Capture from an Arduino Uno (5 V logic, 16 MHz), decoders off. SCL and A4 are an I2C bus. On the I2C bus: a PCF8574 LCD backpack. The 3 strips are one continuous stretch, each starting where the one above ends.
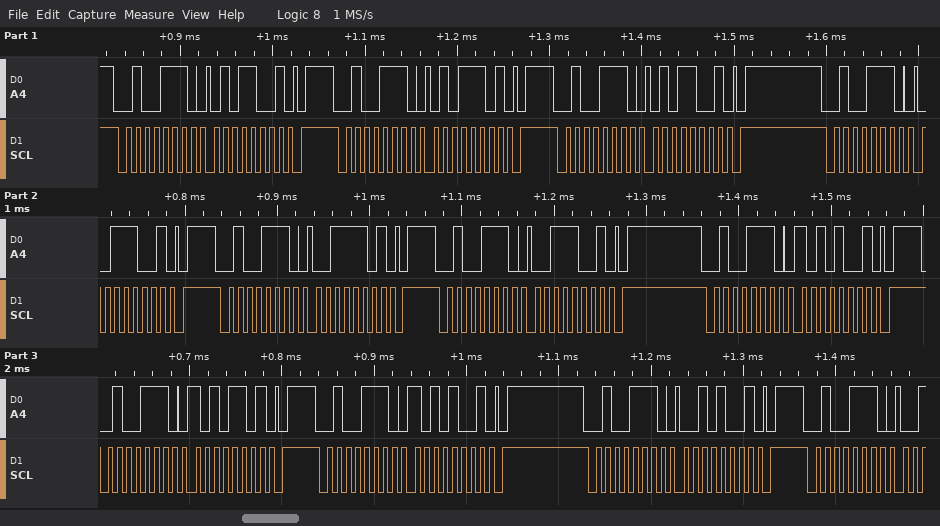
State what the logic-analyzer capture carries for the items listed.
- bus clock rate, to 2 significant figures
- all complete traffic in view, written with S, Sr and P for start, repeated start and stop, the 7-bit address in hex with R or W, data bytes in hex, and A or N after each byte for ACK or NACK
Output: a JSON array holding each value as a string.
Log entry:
["100 kHz", "S 27W A 59 A P S 27W A 5D A P S 27W A 59 A P S 27W A 39 A P S 27W A 3D A P S 27W A 39 A P S 27W A A9 A P S 27W A AD A P S 27W A A9 A P S 27W A 29 A P S 27W A"]
